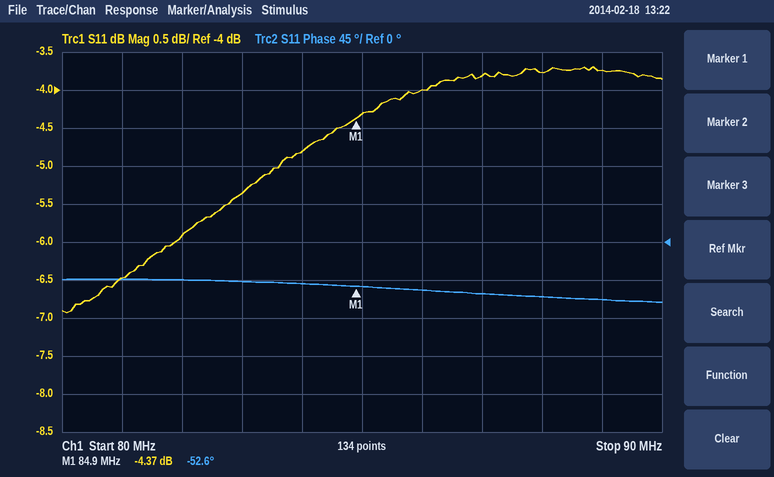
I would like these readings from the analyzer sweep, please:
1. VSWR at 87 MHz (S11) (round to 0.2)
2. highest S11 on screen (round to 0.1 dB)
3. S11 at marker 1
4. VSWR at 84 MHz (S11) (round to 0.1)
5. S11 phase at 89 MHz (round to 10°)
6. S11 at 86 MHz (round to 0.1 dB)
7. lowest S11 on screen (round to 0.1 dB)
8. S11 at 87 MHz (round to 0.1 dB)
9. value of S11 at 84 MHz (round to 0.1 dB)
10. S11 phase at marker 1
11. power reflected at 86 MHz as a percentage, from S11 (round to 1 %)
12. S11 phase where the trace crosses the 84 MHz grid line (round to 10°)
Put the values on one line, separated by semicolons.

4.6; -3.7 dB; -4.37 dB; 3.7; -70°; -4.0 dB; -6.9 dB; -3.8 dB; -4.8 dB; -52.6°; 40 %; -50°
